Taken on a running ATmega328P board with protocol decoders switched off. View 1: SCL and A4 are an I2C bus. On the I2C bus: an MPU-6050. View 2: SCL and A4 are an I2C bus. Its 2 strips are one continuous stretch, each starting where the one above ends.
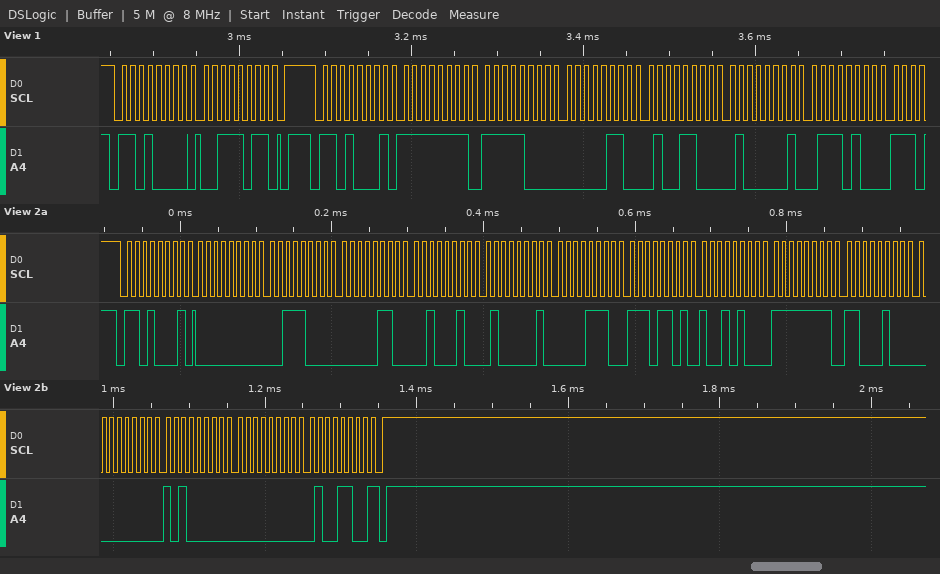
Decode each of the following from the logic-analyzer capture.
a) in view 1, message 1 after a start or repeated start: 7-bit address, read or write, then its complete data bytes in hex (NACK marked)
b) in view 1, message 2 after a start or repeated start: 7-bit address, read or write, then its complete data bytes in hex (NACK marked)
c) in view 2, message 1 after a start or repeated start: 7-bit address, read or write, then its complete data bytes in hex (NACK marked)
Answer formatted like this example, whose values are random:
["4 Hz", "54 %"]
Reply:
["0x68 write: 3B", "0x68 read: FF F8 06 4C 41 74", "0x68 read: 00 38 06 22 41 0E ED 94 FF C4 00 A0 00 4C NACK"]
